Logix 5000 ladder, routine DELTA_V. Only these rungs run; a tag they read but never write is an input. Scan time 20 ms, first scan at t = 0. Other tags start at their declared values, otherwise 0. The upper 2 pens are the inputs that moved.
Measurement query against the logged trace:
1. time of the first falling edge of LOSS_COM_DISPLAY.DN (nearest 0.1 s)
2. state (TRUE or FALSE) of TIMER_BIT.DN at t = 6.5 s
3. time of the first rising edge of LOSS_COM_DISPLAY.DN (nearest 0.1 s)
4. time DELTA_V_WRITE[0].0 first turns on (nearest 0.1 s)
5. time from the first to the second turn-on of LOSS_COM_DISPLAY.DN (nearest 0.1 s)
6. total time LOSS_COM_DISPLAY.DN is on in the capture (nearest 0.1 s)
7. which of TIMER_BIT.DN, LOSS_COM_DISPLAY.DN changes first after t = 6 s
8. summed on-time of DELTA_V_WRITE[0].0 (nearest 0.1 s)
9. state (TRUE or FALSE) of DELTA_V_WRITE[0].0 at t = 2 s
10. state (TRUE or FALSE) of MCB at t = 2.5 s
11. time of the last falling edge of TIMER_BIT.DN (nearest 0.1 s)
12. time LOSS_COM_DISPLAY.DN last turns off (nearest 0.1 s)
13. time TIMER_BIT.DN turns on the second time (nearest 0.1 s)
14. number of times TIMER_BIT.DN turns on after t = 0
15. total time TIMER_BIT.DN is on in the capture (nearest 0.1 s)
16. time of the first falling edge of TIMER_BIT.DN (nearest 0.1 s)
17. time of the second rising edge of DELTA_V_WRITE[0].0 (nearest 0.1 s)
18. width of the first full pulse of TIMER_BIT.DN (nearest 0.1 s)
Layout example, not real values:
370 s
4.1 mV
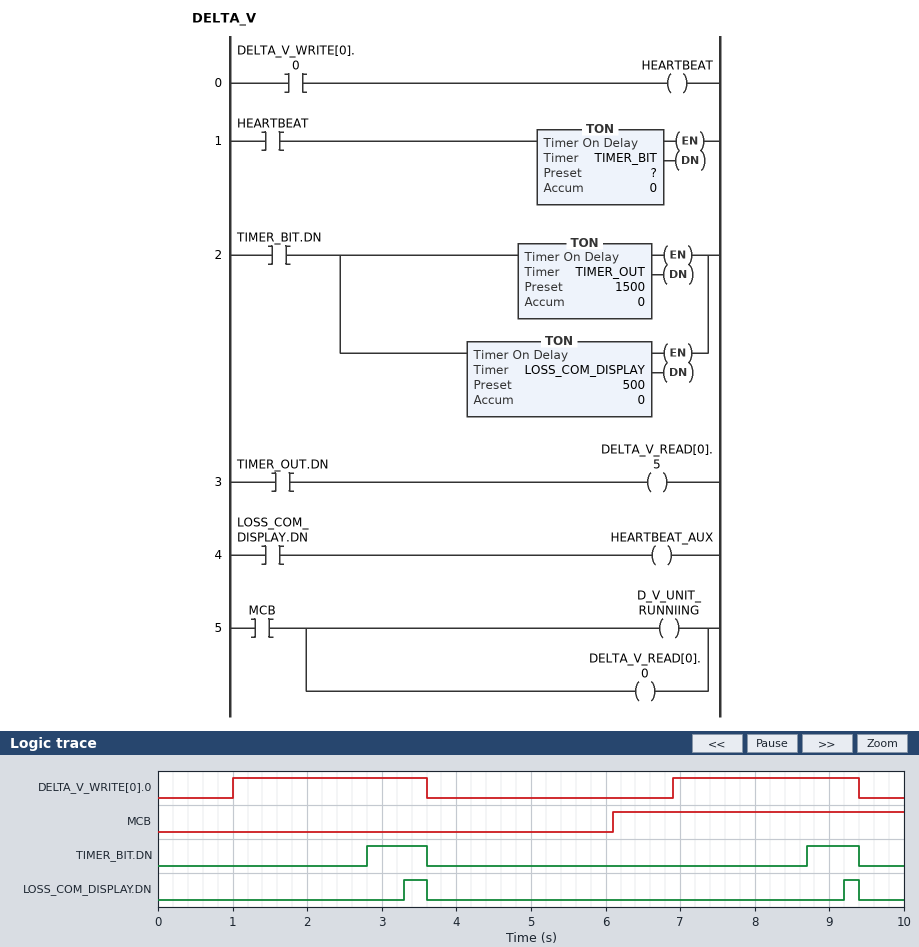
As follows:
3.6 s
FALSE
3.3 s
1.0 s
5.9 s
0.5 s
TIMER_BIT.DN
5.1 s
TRUE
FALSE
9.4 s
9.4 s
8.7 s
2
1.5 s
3.6 s
6.9 s
0.8 s
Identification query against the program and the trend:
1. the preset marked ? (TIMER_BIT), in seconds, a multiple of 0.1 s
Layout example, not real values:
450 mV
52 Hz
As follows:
1.8 s
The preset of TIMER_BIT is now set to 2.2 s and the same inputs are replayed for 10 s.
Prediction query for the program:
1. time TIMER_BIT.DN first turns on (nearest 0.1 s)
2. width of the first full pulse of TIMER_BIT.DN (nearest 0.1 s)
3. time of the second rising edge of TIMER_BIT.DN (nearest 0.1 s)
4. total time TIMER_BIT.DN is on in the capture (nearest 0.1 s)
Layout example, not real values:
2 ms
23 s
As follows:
3.2 s
0.4 s
9.1 s
0.7 s
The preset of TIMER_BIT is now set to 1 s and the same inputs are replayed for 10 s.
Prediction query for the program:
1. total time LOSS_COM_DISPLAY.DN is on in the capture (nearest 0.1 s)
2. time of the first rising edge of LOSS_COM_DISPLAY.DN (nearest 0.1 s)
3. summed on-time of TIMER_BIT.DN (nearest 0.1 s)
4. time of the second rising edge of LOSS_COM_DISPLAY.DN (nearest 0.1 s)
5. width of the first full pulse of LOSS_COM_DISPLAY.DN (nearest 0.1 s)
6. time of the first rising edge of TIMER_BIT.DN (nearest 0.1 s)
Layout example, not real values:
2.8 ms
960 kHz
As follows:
2.1 s
2.5 s
3.1 s
8.4 s
1.1 s
2.0 s
